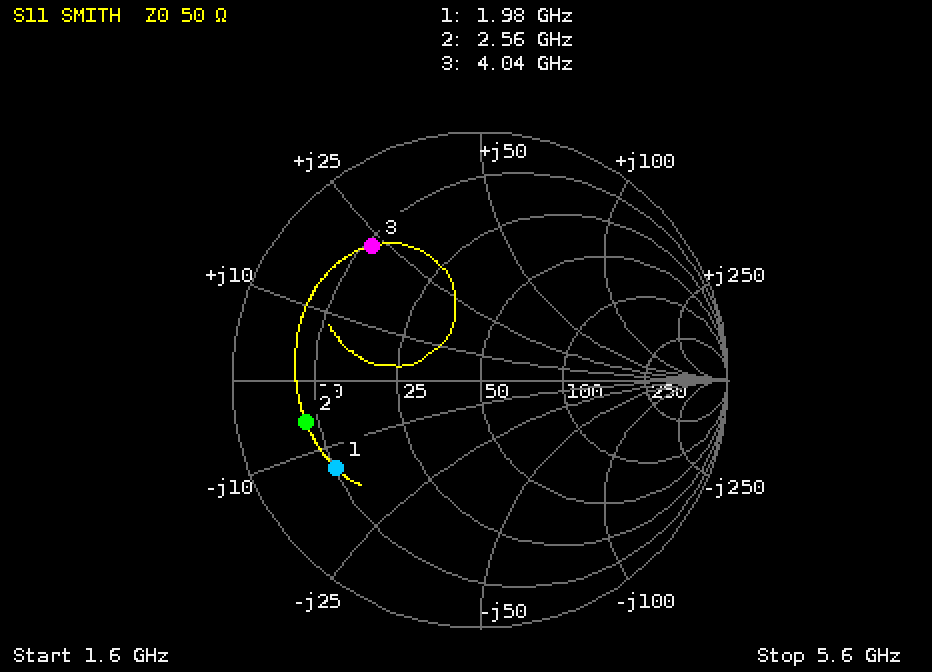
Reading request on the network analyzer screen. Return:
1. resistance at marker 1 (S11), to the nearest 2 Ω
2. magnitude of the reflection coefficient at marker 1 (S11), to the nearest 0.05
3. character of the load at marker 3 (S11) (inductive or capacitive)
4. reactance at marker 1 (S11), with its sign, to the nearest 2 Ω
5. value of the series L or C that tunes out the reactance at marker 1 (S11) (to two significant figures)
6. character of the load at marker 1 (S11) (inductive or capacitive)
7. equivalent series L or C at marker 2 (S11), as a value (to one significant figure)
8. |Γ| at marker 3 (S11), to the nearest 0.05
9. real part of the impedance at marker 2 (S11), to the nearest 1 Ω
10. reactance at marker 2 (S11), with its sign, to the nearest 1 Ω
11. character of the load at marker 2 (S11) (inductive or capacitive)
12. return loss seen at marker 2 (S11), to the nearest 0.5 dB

10 Ω
0.70
inductive
-14 Ω
1.1 nH
capacitive
10 pF
0.70
8 Ω
-6 Ω
capacitive
3.0 dB
